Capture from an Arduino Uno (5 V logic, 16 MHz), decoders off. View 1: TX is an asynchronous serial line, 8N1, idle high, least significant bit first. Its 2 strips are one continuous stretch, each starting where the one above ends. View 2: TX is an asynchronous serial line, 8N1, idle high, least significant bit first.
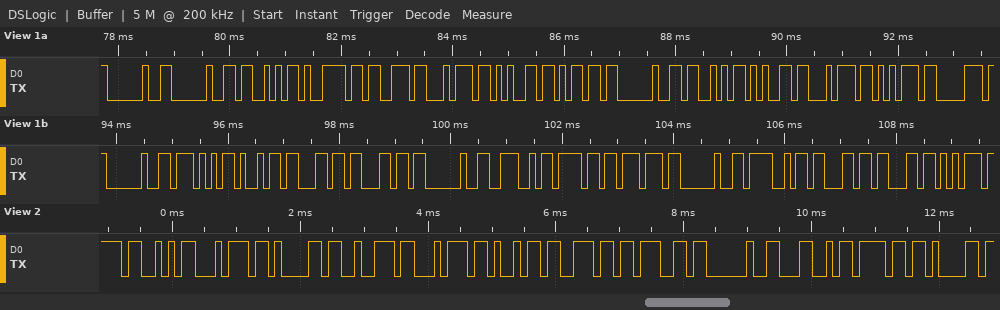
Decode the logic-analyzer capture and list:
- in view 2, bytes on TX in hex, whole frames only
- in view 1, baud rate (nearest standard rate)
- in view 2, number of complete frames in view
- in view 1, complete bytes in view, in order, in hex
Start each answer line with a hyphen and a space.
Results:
- 53 74 61 72 74 69 6E 67 20 4C 6F 61
- 9600 baud
- 12
- 20 20 53 79 73 74 65 6D 20 53 65 74 75 70 20 57 69 6C 6C 20 4E 6F 77 20 4F 63 63 75
